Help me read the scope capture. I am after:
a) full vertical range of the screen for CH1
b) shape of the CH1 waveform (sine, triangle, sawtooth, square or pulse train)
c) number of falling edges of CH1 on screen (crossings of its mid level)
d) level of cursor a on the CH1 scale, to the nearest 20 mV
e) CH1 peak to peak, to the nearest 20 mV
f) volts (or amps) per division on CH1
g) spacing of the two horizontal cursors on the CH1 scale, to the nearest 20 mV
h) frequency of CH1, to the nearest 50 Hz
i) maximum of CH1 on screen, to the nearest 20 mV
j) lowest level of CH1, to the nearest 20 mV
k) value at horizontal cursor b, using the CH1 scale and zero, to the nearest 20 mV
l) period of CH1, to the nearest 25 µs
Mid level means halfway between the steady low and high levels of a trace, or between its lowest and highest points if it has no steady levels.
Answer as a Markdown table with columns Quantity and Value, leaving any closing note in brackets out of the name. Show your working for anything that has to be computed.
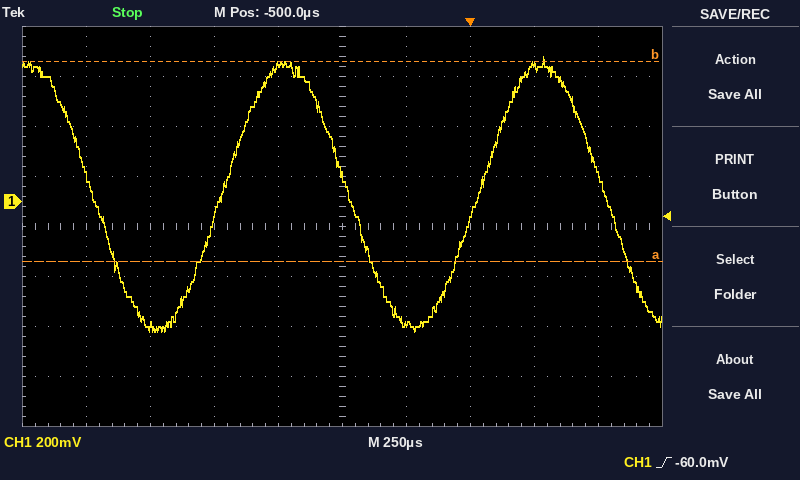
| Quantity | Value |
|---|---|
| full vertical range of the screen for CH1 | 1.6 V |
| shape of the CH1 waveform | sine |
| number of falling edges of CH1 on screen | 3 |
| level of cursor a on the CH1 scale, to the nearest 20 mV | -240 mV |
| CH1 peak to peak, to the nearest 20 mV | 580 mV − (-520 mV) = 1.10 V |
| volts (or amps) per division on CH1 | 200 mV |
| spacing of the two horizontal cursors on the CH1 scale, to the nearest 20 mV | 800 mV |
| frequency of CH1, to the nearest 50 Hz | 1 / 1.000 ms ≈ 1.00 kHz |
| maximum of CH1 on screen, to the nearest 20 mV | 580 mV |
| lowest level of CH1, to the nearest 20 mV | -520 mV |
| value at horizontal cursor b, using the CH1 scale and zero, to the nearest 20 mV | 560 mV |
| period of CH1, to the nearest 25 µs | 1.000 ms |
